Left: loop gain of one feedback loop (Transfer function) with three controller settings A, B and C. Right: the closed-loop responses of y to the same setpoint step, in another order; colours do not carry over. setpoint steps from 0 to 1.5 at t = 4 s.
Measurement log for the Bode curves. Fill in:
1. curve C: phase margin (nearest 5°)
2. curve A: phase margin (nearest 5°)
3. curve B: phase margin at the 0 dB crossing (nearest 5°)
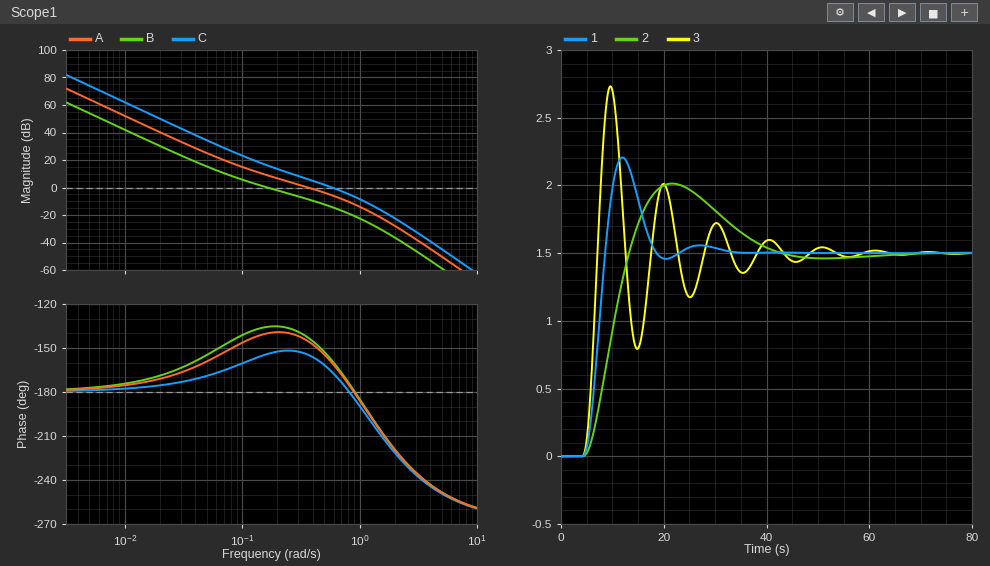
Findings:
15°
35°
45°
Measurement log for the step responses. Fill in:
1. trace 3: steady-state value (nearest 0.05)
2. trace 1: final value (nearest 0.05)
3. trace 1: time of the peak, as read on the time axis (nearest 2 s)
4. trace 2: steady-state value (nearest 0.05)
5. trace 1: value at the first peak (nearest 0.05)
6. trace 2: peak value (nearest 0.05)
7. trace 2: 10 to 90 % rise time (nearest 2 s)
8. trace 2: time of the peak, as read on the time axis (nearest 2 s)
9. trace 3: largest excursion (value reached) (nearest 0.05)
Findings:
1.50
1.50
12 s
1.50
2.20
2.00
6 s
22 s
2.75
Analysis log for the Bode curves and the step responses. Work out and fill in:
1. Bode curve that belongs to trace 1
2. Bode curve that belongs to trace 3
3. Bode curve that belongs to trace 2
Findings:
A
C
B
